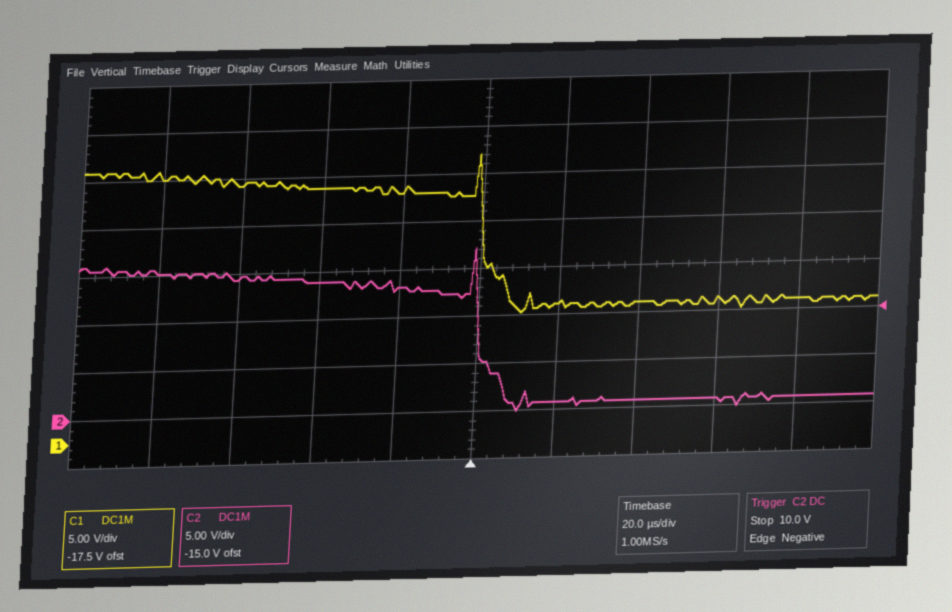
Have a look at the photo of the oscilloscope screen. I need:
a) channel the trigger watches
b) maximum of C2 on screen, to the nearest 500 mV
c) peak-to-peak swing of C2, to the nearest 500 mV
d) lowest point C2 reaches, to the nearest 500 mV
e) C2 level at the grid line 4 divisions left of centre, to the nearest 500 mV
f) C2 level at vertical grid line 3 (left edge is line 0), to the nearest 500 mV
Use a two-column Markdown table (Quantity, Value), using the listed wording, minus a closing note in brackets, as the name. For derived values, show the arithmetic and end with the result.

| Quantity | Value |
|---|---|
| channel the trigger watches | C2 |
| maximum of C2 on screen, to the nearest 500 mV | 17.0 V |
| peak-to-peak swing of C2, to the nearest 500 mV | 17.0 V − (0.0 V) = 17.0 V |
| lowest point C2 reaches, to the nearest 500 mV | 0.0 V |
| C2 level at the grid line 4 divisions left of centre, to the nearest 500 mV | 15.5 V |
| C2 level at vertical grid line 3 (left edge is line 0), to the nearest 500 mV | 14.0 V |
